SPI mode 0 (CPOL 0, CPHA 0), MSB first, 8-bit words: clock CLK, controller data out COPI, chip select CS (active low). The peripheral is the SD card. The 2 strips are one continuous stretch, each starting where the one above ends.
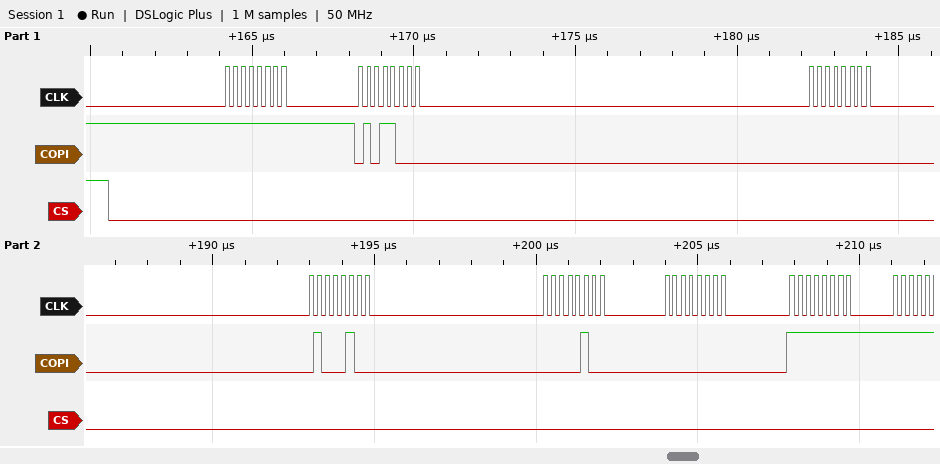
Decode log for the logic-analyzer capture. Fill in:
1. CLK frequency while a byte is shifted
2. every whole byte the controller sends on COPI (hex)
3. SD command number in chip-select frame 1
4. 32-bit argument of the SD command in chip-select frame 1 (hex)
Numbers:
4 MHz
0xFF 0x58 0x00 0x44 0x04 0x00 0xFF
CMD24
0x00440400
